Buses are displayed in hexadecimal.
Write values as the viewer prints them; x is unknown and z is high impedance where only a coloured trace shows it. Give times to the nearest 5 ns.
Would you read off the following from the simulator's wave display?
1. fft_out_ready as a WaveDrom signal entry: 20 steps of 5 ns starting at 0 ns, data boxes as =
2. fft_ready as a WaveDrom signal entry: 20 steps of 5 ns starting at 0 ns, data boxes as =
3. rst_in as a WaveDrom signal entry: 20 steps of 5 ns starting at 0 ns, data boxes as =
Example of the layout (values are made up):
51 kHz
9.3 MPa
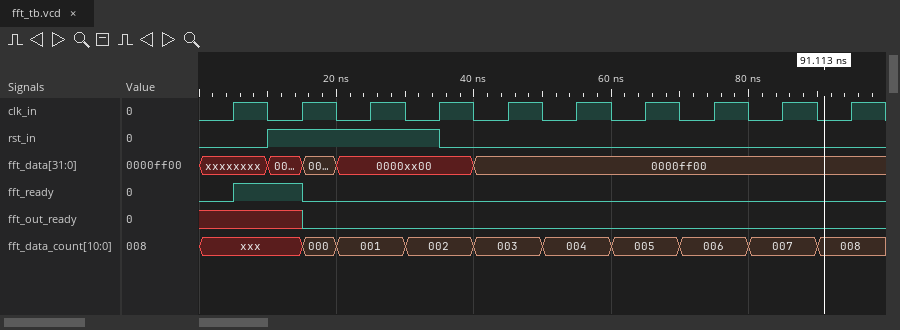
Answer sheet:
{name: 'fft_out_ready', wave: 'x..0................'}
{name: 'fft_ready', wave: '01.0................'}
{name: 'rst_in', wave: '0.1....0............'}
